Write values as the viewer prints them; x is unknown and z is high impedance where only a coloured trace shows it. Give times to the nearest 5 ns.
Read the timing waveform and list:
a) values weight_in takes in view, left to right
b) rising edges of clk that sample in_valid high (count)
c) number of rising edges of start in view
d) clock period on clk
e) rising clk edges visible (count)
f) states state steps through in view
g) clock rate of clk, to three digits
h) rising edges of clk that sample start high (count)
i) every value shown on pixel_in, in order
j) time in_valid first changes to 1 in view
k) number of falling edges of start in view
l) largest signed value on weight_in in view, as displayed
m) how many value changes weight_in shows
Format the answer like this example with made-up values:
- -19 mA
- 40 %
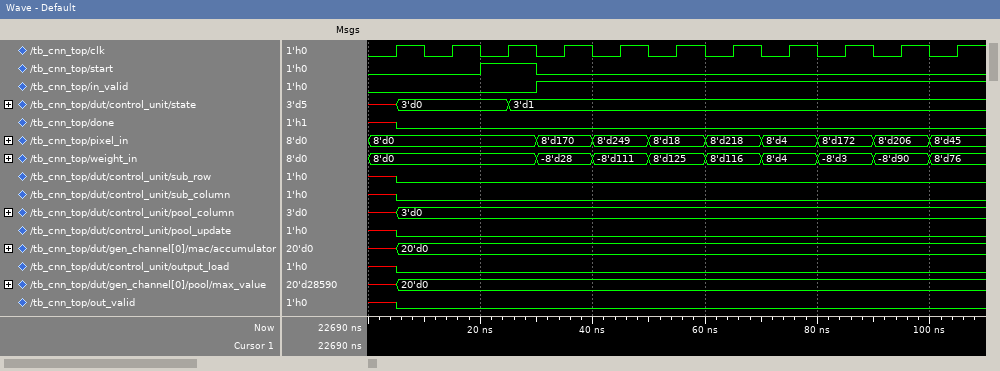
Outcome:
- 8'd0, -8'd28, -8'd111, 8'd125, 8'd116, 8'd4, -8'd3, -8'd90, 8'd76
- 8
- 1
- 10 ns
- 11
- x, 3'd0, 3'd1
- 100 MHz
- 1
- 8'd0, 8'd170, 8'd249, 8'd18, 8'd218, 8'd4, 8'd172, 8'd206, 8'd45
- 30 ns
- 1
- 8'd125
- 8
